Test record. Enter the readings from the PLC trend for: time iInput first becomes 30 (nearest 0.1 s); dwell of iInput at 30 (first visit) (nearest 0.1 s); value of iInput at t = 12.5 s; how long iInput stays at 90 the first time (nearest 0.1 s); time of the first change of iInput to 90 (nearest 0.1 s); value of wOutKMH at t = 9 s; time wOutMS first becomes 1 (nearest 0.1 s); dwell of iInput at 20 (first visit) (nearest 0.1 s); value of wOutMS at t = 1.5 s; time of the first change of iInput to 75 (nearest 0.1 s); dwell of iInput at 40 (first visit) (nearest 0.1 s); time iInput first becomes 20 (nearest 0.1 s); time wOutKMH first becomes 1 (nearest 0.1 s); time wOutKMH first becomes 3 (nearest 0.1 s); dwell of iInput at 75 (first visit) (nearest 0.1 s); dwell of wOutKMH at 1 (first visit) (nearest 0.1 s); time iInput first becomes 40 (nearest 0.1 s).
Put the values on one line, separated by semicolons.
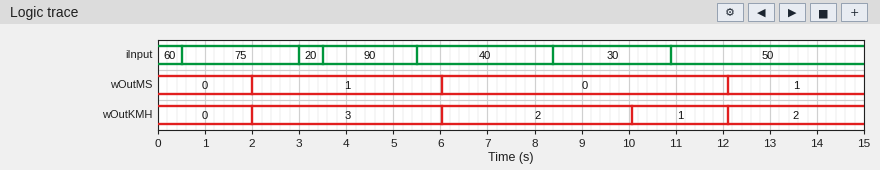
8.4 s; 2.5 s; 50; 2.0 s; 3.5 s; 2; 2.0 s; 0.5 s; 0; 0.5 s; 2.9 s; 3.0 s; 10.1 s; 2.0 s; 2.5 s; 2.0 s; 5.5 s
